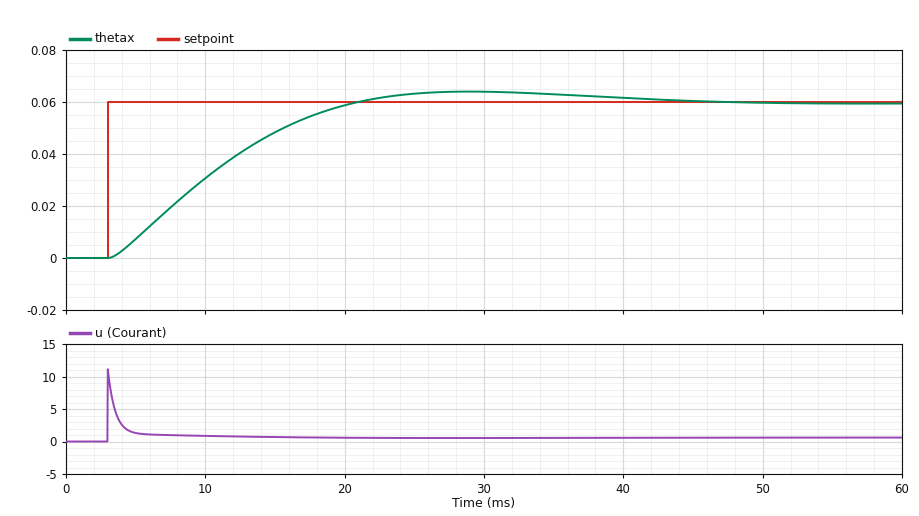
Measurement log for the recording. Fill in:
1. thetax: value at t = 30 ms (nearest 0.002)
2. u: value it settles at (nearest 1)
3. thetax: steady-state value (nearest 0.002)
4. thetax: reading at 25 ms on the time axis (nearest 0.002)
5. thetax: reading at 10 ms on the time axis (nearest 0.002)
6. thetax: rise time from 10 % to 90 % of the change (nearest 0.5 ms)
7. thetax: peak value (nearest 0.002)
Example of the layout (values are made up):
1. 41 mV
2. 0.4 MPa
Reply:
1. 0.064
2. 1
3. 0.060
4. 0.064
5. 0.030
6. 12.5 ms
7. 0.064
